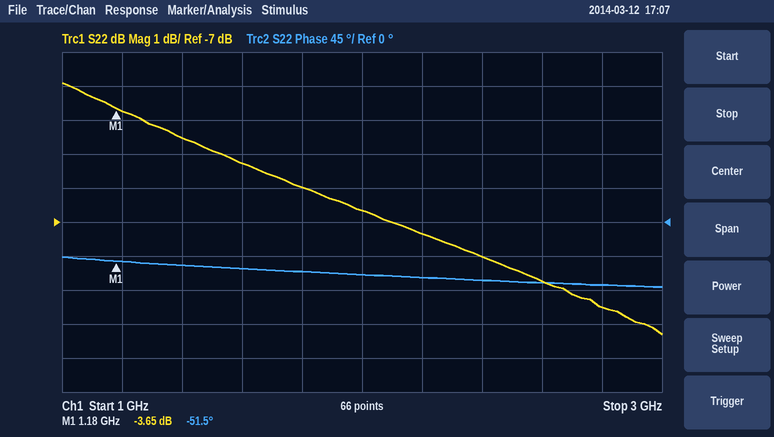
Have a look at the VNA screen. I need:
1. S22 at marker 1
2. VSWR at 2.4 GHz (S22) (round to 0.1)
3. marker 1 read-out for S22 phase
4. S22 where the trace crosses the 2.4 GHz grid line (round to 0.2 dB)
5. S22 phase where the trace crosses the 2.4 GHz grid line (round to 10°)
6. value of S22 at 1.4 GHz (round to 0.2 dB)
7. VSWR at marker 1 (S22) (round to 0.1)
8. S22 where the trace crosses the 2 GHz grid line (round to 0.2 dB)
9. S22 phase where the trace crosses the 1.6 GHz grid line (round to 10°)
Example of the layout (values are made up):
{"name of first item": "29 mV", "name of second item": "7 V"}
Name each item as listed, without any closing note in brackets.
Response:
{"S22 at marker 1": "-3.65 dB", "VSWR at 2.4 GHz (S22)": "2.3", "marker 1 read-out for S22 phase": "-51.5°", "S22 where the trace crosses the 2.4 GHz grid line": "-8.0 dB", "S22 phase where the trace crosses the 2.4 GHz grid line": "-80°", "value of S22 at 1.4 GHz": "-4.6 dB", "VSWR at marker 1 (S22)": "4.8", "S22 where the trace crosses the 2 GHz grid line": "-6.6 dB", "S22 phase where the trace crosses the 1.6 GHz grid line": "-60°"}
